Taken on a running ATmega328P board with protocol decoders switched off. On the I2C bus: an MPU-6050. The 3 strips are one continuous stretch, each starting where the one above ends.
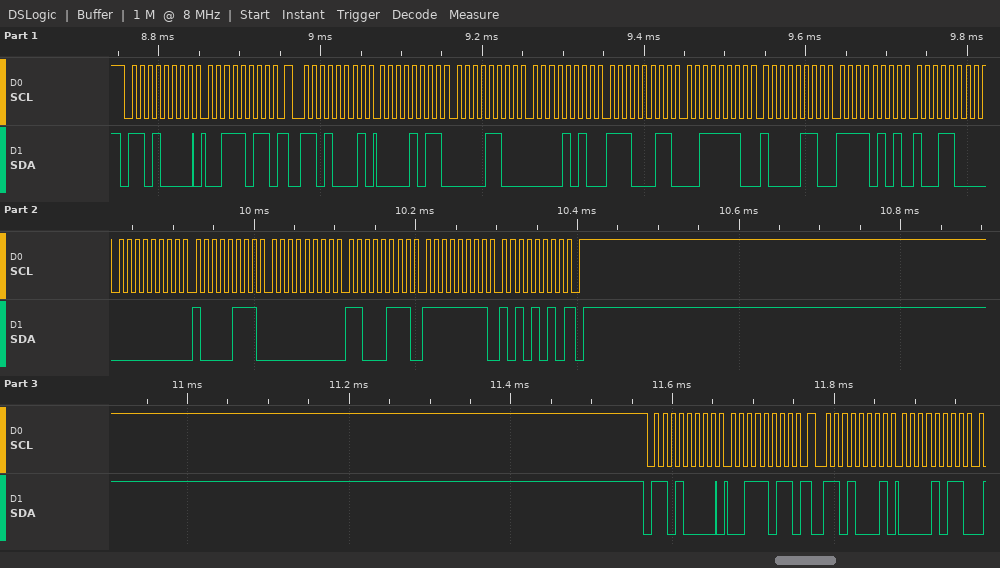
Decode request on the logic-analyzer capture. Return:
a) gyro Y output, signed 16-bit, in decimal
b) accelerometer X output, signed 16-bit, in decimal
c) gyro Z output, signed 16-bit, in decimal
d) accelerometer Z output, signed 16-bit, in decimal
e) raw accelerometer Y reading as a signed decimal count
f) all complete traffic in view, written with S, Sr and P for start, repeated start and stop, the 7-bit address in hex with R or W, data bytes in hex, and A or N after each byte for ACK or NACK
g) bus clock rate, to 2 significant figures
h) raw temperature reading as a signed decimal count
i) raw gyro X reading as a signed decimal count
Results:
199
2828
-86
16006
2787
S 68W A 3B A Sr 68R A 0B A 0C A 0A A E3 A 3E A 86 A F5 A 98 A 00 A 87 A 00 A C7 A FF A AA N P S 68W A 3B A Sr 68R A 0B A
100 kHz
-2664
135
